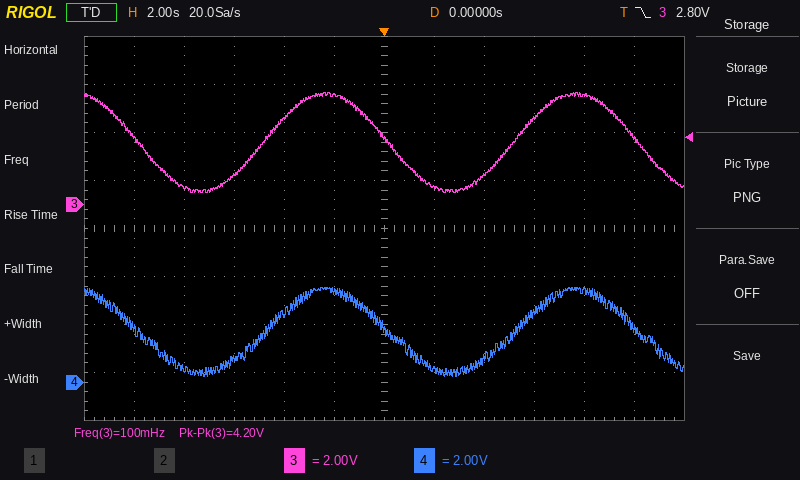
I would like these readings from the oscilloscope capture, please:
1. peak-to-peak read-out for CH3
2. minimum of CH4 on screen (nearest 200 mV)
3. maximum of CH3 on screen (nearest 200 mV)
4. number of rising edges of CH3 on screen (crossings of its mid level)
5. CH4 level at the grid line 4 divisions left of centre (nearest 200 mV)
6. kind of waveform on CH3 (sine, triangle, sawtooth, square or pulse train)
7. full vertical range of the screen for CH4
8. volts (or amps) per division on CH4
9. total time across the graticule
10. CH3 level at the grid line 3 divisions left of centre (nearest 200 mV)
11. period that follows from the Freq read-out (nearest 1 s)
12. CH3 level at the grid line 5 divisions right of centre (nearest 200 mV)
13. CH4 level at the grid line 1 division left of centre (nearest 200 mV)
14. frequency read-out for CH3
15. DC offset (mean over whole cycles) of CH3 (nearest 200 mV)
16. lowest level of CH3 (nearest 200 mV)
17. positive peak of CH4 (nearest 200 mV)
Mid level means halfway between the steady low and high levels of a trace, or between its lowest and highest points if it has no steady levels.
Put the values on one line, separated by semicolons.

4.20 V; 200 mV; 4.6 V; 2; 600 mV; sine; 16 V; 2 V; 24 s; 1.2 V; 10 s; 2.8 V; 3.8 V; 100 mHz; 2.6 V; 400 mV; 4.0 V
